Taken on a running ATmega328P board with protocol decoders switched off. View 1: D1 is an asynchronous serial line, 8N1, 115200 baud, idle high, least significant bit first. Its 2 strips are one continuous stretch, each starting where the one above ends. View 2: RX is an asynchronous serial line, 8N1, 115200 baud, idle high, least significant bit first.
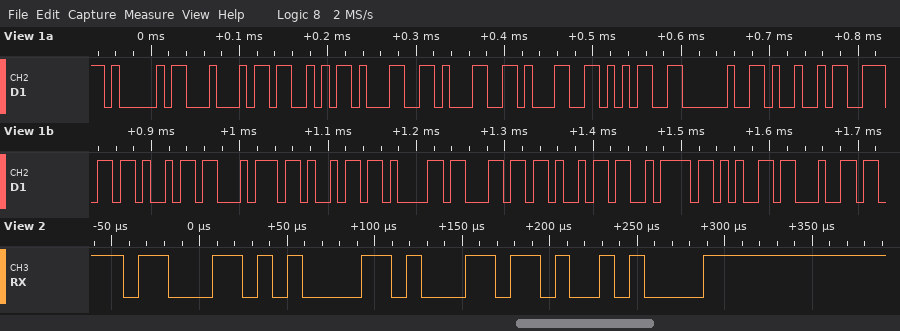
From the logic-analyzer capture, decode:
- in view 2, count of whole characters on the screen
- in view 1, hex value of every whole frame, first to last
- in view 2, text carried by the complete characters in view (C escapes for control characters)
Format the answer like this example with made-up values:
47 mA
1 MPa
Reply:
4
41 44 53 31 31 31 35 20 49 6E 69 74 69 61 6C 69 7A 65 64
"cal\n"
